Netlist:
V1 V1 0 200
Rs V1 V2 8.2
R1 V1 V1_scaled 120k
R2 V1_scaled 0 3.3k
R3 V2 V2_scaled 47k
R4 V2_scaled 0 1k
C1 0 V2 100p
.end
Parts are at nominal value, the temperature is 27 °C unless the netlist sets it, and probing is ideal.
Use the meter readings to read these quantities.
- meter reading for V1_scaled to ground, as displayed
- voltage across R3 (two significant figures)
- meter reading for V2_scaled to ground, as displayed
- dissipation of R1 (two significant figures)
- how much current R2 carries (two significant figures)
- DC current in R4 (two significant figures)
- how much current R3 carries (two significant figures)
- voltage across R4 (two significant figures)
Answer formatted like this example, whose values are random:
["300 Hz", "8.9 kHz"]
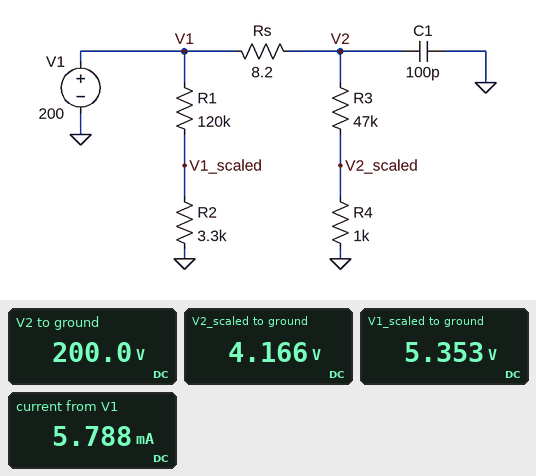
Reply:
["5.353 V", "200 V", "4.166 V", "320 mW", "1.6 mA", "4.2 mA", "4.2 mA", "4.2 V"]
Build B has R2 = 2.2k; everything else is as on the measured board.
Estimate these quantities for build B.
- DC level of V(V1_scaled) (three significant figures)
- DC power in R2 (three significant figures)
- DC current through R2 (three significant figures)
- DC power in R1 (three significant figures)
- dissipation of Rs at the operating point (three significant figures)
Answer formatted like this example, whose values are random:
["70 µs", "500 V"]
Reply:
["3.60 V", "5.89 mW", "1.64 mA", "321 mW", "142 µW"]
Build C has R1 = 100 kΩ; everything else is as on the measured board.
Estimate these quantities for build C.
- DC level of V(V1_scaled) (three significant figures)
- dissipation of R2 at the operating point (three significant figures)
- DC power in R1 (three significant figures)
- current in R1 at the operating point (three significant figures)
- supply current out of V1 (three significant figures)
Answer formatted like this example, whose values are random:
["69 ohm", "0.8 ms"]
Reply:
["6.39 V", "12.4 mW", "375 mW", "1.94 mA", "6.10 mA"]
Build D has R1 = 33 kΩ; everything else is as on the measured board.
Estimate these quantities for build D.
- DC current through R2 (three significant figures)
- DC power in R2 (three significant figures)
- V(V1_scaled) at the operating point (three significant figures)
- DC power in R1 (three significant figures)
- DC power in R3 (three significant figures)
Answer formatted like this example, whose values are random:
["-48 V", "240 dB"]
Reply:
["5.51 mA", "100 mW", "18.2 V", "1.00 W", "816 mW"]
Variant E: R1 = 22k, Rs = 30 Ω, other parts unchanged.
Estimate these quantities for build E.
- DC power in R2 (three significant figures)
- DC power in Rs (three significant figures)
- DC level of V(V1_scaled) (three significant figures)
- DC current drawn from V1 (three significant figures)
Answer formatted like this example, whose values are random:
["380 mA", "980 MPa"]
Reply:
["206 mW", "520 µW", "26.1 V", "12.1 mA"]
